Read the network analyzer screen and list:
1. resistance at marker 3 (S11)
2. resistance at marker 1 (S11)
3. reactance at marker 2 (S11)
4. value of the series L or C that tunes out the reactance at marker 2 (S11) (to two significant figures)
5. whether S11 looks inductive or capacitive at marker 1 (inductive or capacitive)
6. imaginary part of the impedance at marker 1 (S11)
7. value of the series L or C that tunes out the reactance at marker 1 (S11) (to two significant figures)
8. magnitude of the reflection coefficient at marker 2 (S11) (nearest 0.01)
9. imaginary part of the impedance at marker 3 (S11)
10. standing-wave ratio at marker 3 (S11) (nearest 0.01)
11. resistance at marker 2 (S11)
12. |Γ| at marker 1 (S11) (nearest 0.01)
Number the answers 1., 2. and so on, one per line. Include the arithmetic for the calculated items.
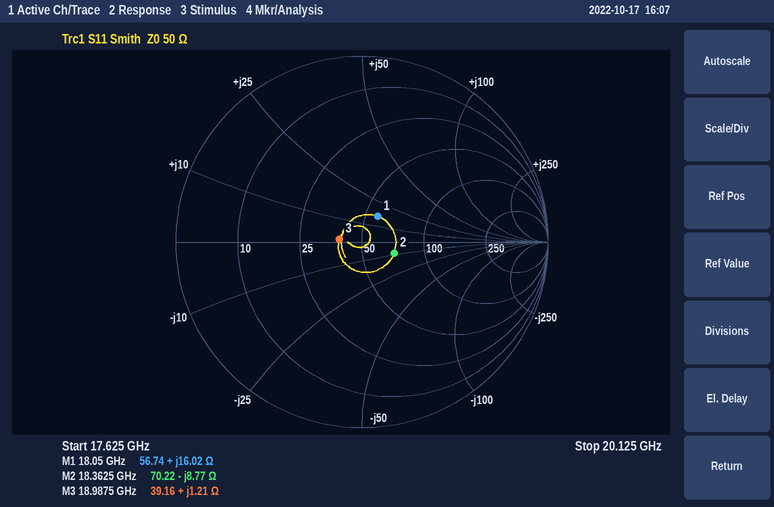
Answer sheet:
1. 39.16 Ω
2. 56.74 Ω
3. -8.77 Ω
4. L = 8.77 Ω/(2π × 18.3625 GHz) ≈ 76 pH
5. inductive
6. +16.02 Ω
7. C = 1/(2π × 18.05 GHz × 16.02 Ω) ≈ 550 fF
8. 0.18
9. +1.21 Ω
10. 1.28
11. 70.22 Ω
12. 0.16
